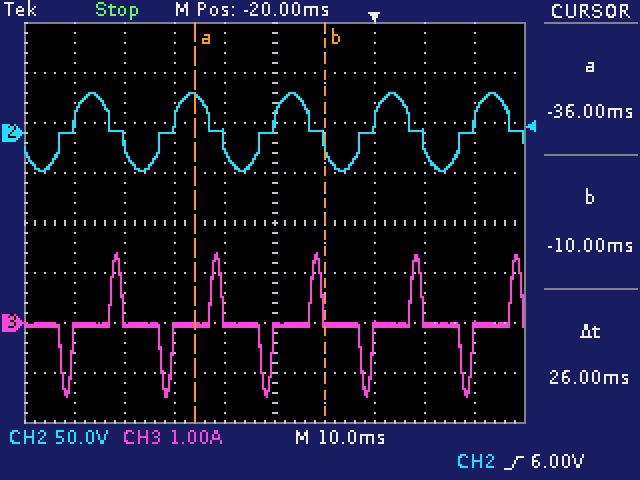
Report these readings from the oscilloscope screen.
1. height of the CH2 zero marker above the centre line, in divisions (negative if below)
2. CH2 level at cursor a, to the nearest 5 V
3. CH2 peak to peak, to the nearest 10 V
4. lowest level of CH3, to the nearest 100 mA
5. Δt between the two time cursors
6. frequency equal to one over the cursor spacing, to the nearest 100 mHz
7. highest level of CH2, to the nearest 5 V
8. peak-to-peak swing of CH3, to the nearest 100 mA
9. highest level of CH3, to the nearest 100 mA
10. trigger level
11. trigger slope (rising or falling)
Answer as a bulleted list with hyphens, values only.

- +1.8 div
- 35 V
- 80 V
- -1.5 A
- 26 ms
- 38.5 Hz
- 40 V
- 2.9 A
- 1.4 A
- 6.00 V
- rising
